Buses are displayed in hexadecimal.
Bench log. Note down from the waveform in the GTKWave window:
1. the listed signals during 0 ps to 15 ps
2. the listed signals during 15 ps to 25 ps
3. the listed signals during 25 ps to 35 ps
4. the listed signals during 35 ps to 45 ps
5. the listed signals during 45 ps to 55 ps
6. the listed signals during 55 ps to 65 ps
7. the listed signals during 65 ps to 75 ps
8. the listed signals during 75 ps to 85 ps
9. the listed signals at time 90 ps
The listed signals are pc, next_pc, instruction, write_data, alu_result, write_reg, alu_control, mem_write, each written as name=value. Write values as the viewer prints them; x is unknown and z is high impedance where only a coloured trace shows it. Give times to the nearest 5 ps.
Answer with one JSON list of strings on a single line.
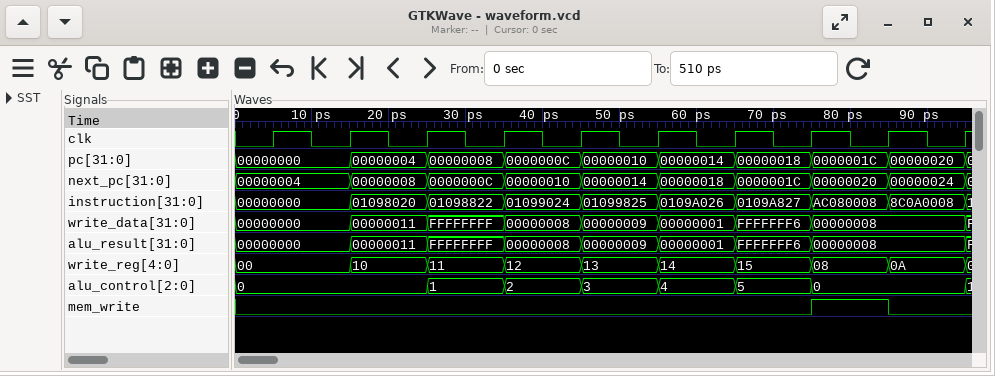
["pc=00000000, next_pc=00000004, instruction=00000000, write_data=00000000, alu_result=00000000, write_reg=00, alu_control=0, mem_write=0", "pc=00000004, next_pc=00000008, instruction=01098020, write_data=00000011, alu_result=00000011, write_reg=10, alu_control=0, mem_write=0", "pc=00000008, next_pc=0000000C, instruction=01098822, write_data=FFFFFFFF, alu_result=FFFFFFFF, write_reg=11, alu_control=1, mem_write=0", "pc=0000000C, next_pc=00000010, instruction=01099024, write_data=00000008, alu_result=00000008, write_reg=12, alu_control=2, mem_write=0", "pc=00000010, next_pc=00000014, instruction=01099825, write_data=00000009, alu_result=00000009, write_reg=13, alu_control=3, mem_write=0", "pc=00000014, next_pc=00000018, instruction=0109A026, write_data=00000001, alu_result=00000001, write_reg=14, alu_control=4, mem_write=0", "pc=00000018, next_pc=0000001C, instruction=0109A827, write_data=FFFFFFF6, alu_result=FFFFFFF6, write_reg=15, alu_control=5, mem_write=0", "pc=0000001C, next_pc=00000020, instruction=AC080008, write_data=00000008, alu_result=00000008, write_reg=08, alu_control=0, mem_write=1", "pc=00000020, next_pc=00000024, instruction=8C0A0008, write_data=00000008, alu_result=00000008, write_reg=0A, alu_control=0, mem_write=0"]
